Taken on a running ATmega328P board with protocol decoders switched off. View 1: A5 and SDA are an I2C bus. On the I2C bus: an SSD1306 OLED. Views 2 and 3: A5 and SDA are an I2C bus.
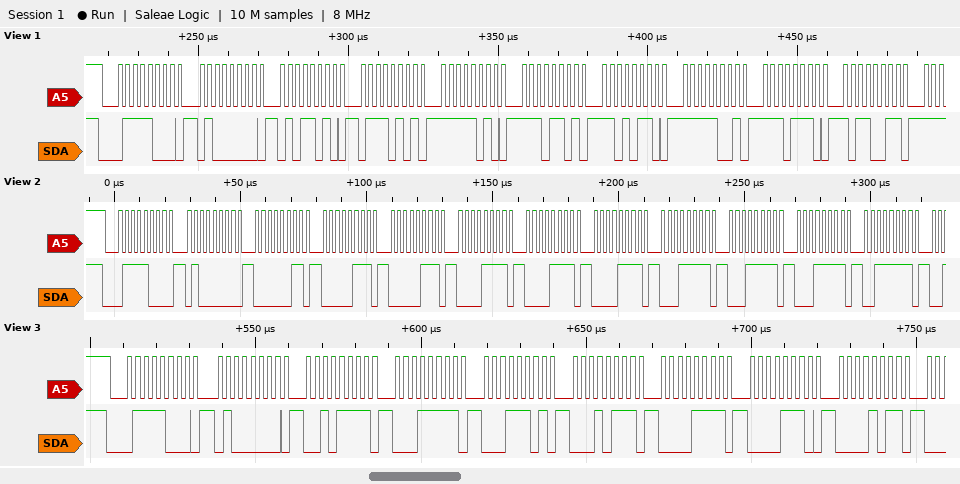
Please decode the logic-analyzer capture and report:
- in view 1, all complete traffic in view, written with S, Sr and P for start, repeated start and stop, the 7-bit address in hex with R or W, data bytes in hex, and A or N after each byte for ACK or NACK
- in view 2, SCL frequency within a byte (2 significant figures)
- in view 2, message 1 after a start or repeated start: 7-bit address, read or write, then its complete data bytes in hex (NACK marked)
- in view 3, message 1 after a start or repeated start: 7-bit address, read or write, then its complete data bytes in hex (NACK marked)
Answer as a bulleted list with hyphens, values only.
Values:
- S 3CW A 40 A 5A A 75 A FA A ED A D6 A F9 A EE A B3 A
- 400 kHz
- 0x3C write: 40 03 07 07 0F 0F 0F 1F 1F 1F 3F
- 0x3C write: 40 2F 1F 1D 17 0F 0E 0B
